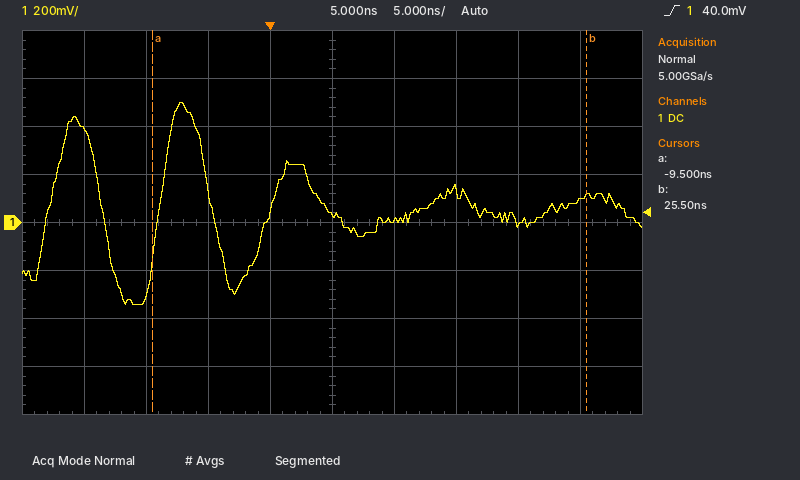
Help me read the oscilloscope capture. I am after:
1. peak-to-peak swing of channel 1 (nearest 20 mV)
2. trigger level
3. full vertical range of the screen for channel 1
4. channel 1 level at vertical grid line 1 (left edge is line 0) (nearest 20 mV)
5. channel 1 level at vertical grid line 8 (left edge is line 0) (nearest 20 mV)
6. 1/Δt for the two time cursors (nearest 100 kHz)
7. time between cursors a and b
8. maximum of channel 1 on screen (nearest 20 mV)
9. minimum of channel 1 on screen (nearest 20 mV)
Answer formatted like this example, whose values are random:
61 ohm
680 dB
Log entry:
840 mV
40.0 mV
1.6 V
380 mV
0 mV
28.6 MHz
35.0 ns
500 mV
-340 mV
